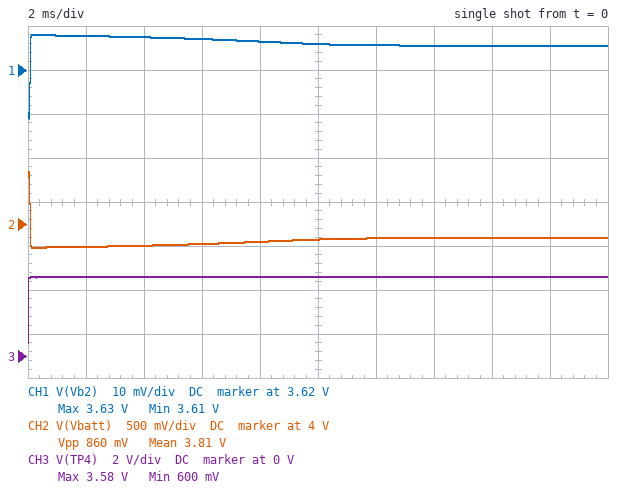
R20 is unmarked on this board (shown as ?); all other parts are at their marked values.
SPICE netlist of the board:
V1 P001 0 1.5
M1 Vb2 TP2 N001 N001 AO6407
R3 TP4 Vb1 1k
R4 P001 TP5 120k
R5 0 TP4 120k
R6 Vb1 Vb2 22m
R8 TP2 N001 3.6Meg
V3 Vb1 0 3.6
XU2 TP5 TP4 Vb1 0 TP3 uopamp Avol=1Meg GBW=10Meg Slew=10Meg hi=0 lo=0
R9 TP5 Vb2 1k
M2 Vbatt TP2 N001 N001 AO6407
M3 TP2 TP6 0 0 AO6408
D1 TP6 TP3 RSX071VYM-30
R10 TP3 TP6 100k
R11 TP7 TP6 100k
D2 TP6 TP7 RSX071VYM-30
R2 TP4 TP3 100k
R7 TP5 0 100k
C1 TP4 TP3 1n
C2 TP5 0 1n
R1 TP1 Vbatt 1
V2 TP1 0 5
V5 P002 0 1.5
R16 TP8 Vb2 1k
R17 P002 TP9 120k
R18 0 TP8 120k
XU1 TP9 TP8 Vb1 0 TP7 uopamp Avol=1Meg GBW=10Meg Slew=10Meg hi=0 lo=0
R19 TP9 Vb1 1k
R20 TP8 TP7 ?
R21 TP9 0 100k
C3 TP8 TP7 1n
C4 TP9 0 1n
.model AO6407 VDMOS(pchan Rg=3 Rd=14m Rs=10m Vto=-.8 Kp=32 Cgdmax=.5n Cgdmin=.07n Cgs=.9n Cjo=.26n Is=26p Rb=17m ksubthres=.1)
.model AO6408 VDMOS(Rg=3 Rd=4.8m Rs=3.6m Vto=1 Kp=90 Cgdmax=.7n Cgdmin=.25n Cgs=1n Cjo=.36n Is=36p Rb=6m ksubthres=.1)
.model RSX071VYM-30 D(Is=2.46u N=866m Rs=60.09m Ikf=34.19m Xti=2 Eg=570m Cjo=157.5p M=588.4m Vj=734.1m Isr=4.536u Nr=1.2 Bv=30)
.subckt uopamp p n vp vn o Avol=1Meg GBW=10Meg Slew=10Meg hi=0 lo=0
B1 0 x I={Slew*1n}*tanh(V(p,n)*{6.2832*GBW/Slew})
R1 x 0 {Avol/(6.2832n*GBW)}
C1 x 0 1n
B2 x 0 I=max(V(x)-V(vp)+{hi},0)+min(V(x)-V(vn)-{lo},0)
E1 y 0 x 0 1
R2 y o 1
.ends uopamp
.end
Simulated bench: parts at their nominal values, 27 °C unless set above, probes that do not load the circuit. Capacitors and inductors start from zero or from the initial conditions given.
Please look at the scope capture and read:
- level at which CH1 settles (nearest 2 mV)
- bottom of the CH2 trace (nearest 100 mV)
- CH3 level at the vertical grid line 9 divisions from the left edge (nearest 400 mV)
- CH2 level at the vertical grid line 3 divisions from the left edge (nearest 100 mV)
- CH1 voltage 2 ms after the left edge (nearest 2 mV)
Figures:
3.626 V
3.7 V
3.6 V
3.8 V
3.628 V
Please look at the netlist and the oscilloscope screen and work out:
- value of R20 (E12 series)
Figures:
68 kΩ
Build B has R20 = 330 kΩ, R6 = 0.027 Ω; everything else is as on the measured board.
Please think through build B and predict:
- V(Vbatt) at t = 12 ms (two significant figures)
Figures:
5.0 V
